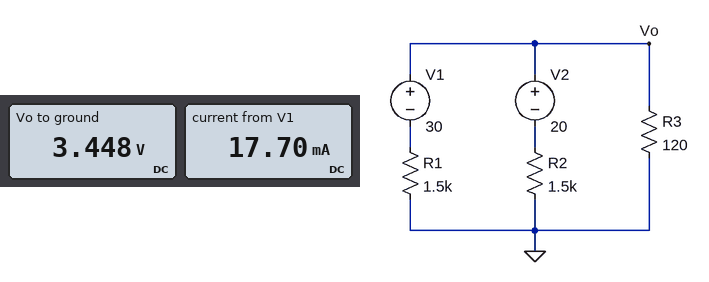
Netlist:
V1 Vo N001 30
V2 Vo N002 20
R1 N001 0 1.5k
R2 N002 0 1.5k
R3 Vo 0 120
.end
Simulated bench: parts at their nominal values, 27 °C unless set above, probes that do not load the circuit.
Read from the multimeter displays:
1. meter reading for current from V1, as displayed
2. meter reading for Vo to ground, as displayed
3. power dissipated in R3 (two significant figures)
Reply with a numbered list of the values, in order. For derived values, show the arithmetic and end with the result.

1. 17.70 mA
2. 3.448 V
3. (3.448 V)^2 / 120 Ω = 99 mW
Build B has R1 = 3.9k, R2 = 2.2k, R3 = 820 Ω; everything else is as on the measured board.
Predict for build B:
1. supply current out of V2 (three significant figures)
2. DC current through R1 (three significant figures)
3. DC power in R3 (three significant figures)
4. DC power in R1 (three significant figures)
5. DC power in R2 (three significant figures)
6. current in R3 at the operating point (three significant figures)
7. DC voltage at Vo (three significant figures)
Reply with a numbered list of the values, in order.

1. 5.14 mA
2. 5.46 mA
3. 92.2 mW
4. 116 mW
5. 58.1 mW
6. 10.6 mA
7. 8.69 V
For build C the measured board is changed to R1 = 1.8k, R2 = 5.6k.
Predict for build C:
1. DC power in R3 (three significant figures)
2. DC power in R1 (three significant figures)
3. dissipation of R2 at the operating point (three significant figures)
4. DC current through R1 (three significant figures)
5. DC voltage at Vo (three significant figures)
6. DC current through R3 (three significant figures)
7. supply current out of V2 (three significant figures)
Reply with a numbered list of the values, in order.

1. 41.5 mW
2. 428 mW
3. 56.4 mW
4. 15.4 mA
5. 2.23 V
6. 18.6 mA
7. 3.17 mA
